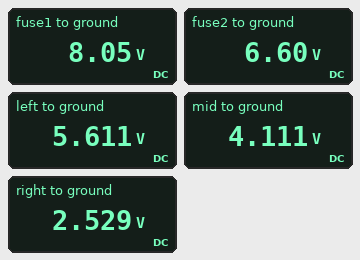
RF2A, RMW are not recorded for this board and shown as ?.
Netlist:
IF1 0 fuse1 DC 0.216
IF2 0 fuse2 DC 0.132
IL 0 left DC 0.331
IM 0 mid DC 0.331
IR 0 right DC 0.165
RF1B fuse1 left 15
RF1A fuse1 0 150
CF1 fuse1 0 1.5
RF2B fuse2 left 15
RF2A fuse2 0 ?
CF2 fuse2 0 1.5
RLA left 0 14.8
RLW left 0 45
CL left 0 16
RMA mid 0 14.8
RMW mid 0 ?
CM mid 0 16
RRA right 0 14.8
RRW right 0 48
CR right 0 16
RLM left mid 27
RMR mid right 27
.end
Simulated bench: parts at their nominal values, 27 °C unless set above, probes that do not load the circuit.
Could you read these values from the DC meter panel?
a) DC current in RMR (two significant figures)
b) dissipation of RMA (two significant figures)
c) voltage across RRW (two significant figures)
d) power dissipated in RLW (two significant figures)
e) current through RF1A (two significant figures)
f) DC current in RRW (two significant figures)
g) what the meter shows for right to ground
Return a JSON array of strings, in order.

["59 mA", "1.1 W", "2.5 V", "700 mW", "54 mA", "53 mA", "2.529 V"]
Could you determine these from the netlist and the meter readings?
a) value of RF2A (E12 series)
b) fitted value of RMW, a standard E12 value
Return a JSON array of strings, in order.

["100 Ω", "82 Ω"]
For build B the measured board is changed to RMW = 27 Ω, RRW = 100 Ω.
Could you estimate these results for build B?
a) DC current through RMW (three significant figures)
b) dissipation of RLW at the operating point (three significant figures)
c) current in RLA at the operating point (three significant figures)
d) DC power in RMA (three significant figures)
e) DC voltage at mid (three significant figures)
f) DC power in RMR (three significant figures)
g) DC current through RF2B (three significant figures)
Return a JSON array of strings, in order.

["130 mA", "661 mW", "369 mA", "836 mW", "3.52 V", "32.8 mW", "67.3 mA"]
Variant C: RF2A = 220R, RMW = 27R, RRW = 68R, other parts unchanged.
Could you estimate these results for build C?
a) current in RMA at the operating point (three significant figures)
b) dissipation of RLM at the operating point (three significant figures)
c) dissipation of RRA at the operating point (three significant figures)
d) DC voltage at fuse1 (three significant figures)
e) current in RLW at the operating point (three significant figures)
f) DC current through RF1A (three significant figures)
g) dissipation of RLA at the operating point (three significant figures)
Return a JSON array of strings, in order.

["240 mA", "172 mW", "417 mW", "8.13 V", "127 mA", "54.2 mA", "2.20 W"]
